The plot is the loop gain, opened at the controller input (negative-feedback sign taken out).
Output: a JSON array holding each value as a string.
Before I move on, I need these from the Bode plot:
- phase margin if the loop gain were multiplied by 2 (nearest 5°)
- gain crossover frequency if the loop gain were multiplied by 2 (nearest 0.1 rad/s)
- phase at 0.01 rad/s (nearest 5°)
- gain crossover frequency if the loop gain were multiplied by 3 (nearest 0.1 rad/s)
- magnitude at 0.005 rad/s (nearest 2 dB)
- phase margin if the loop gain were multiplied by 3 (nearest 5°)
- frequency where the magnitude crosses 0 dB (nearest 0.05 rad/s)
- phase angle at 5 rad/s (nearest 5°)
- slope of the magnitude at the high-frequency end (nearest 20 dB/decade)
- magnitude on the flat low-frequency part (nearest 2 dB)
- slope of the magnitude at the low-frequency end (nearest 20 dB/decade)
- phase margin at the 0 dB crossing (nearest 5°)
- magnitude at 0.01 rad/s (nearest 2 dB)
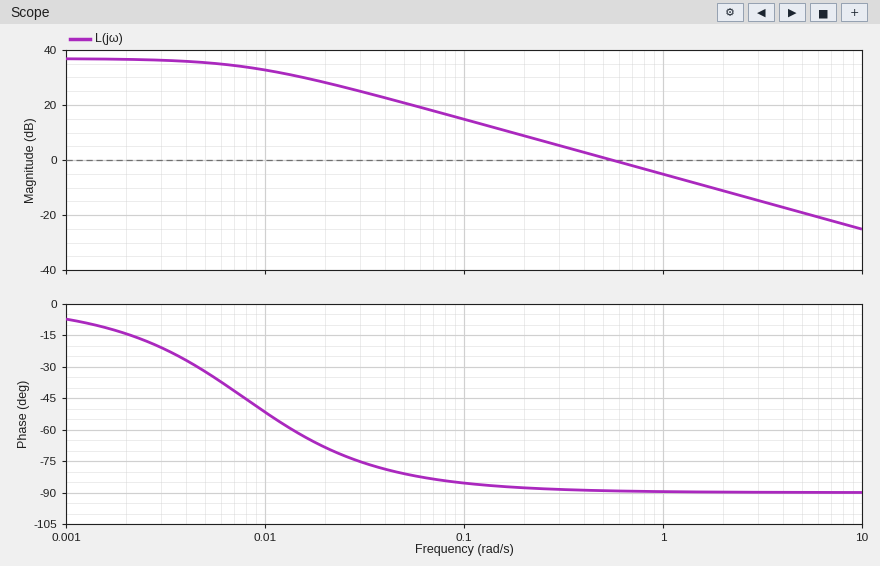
["90°", "1.1 rad/s", "-50°", "1.7 rad/s", "36 dB", "90°", "0.55 rad/s", "-90°", "-20 dB/decade", "36 dB", "0 dB/decade", "90°", "32 dB"]
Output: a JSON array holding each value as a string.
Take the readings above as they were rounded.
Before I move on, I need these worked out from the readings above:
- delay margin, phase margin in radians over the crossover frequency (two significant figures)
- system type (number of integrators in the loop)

["2.9 s", "0"]
